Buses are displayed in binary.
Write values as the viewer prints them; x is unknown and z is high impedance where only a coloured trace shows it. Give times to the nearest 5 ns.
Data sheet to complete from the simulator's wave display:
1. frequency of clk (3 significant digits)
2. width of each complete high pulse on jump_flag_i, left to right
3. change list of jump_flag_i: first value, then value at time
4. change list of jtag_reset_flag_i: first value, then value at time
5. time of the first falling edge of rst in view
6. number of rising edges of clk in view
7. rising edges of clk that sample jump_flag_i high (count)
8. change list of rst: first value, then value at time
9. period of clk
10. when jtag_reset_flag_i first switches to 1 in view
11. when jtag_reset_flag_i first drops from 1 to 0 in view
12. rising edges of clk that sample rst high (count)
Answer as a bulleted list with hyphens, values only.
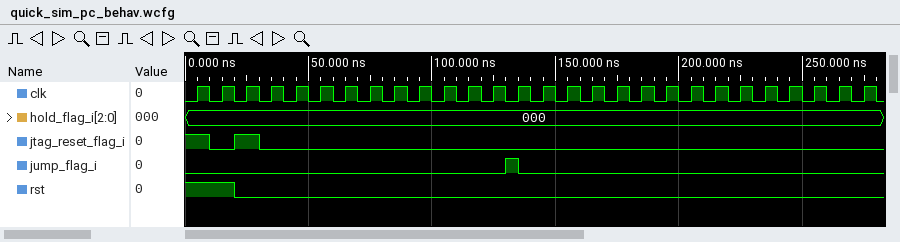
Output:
- 100 MHz
- 5 ns
- 0, 1 at 130 ns, 0 at 135 ns
- 1, 0 at 10 ns, 1 at 20 ns, 0 at 30 ns
- 20 ns
- 28
- 1
- 1, 0 at 20 ns
- 10 ns
- 20 ns
- 10 ns
- 2
